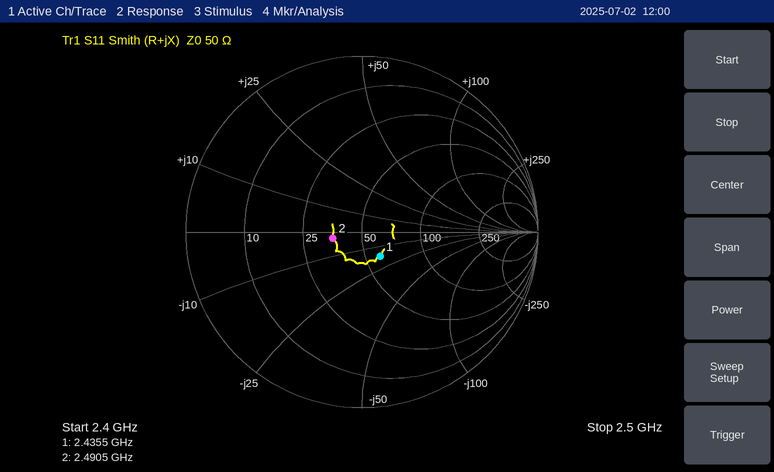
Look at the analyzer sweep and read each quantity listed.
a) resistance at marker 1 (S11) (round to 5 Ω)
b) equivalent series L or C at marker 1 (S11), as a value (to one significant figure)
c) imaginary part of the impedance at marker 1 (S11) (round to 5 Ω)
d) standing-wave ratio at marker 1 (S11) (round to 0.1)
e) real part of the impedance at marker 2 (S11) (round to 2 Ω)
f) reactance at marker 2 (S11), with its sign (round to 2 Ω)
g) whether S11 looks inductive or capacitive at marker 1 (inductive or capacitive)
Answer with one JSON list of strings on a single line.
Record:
["60 Ω", "4 pF", "-15 Ω", "1.4", "36 Ω", "-2 Ω", "capacitive"]
